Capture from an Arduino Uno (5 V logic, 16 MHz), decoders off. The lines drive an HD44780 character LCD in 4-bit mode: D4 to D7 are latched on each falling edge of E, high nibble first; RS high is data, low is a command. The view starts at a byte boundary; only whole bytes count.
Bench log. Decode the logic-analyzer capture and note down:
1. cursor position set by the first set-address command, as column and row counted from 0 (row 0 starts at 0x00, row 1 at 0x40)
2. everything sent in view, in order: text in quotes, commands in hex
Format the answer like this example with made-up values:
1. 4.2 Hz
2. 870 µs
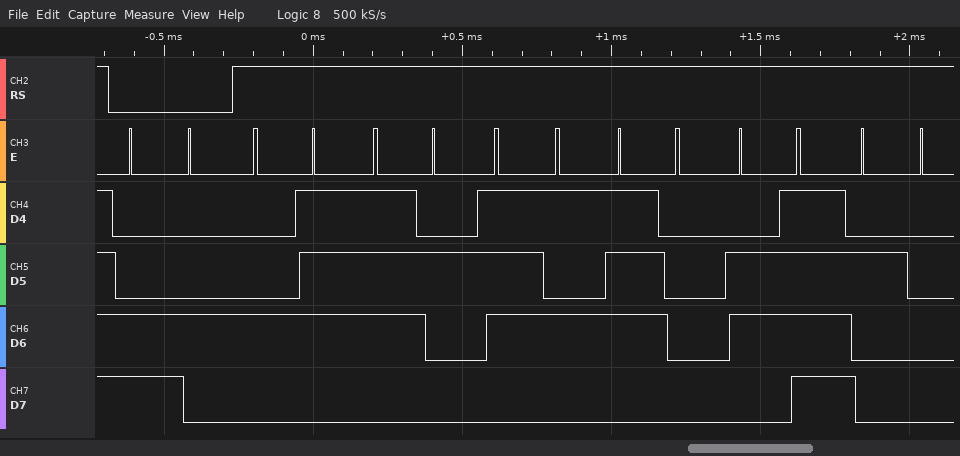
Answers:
1. column 4, row 1
2. 0xC4 "Grupo "
